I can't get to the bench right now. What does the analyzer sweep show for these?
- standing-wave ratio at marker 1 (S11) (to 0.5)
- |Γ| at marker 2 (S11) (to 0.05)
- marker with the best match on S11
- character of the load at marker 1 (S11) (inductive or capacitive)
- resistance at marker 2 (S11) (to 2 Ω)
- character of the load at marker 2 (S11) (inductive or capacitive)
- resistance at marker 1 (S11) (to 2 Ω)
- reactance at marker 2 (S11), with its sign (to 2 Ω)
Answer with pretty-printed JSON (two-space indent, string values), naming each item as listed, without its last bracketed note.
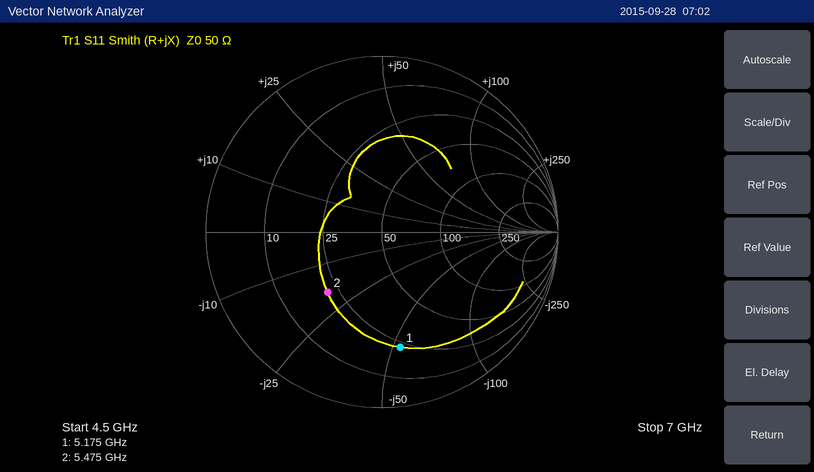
{
  "standing-wave ratio at marker 1 (S11)": "5.0",
  "|Γ| at marker 2 (S11)": "0.45",
  "marker with the best match on S11": "marker 2",
  "character of the load at marker 1 (S11)": "capacitive",
  "resistance at marker 2 (S11)": "22 Ω",
  "character of the load at marker 2 (S11)": "capacitive",
  "resistance at marker 1 (S11)": "22 Ω",
  "reactance at marker 2 (S11), with its sign": "-18 Ω"
}
